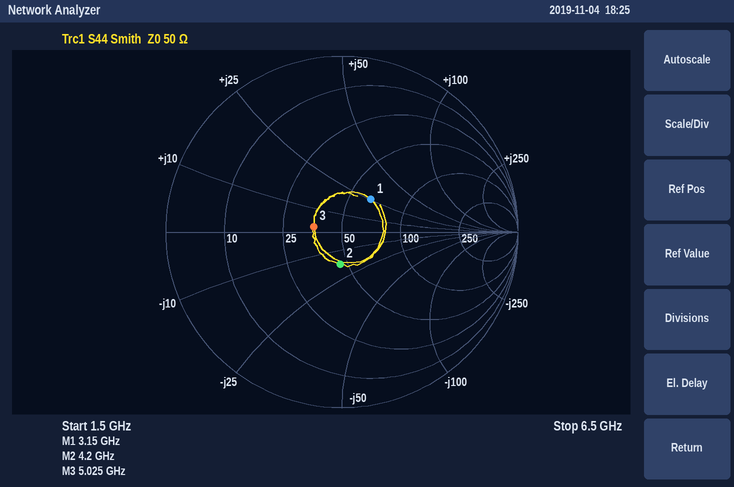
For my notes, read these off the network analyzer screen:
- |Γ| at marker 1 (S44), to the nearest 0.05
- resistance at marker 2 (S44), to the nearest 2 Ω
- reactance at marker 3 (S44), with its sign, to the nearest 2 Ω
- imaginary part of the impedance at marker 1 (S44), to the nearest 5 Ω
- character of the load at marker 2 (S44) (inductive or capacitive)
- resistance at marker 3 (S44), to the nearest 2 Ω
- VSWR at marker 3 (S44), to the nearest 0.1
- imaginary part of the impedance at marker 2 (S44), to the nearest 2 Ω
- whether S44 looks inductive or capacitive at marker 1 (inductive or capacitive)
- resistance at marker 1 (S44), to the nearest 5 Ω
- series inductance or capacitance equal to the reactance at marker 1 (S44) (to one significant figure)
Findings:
0.25
46 Ω
+2 Ω
+25 Ω
capacitive
36 Ω
1.4
-18 Ω
inductive
65 Ω
1 nH
